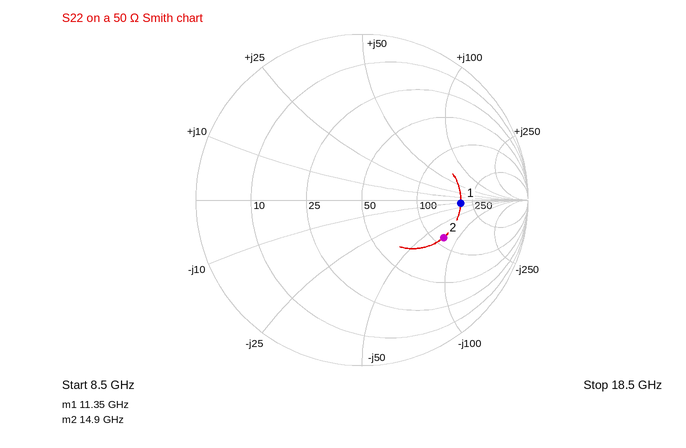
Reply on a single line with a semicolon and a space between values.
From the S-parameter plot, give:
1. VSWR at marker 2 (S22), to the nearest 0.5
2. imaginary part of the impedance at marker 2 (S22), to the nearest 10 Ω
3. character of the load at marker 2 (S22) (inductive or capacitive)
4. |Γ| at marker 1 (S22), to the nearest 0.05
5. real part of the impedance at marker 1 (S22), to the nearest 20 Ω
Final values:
3.5; -70 Ω; capacitive; 0.60; 200 Ω
